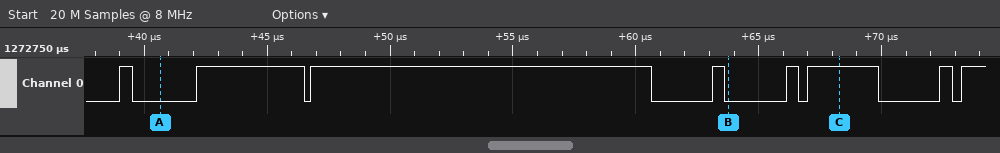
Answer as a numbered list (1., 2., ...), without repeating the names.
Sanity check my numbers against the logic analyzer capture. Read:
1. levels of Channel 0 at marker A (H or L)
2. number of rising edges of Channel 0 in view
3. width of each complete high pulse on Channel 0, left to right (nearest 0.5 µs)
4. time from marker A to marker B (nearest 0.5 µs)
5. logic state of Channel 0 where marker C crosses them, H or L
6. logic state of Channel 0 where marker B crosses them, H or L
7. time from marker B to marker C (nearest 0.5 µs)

1. Channel 0=L
2. 8
3. 0.5 µs, 4.5 µs, 14 µs, 0.5 µs, 0.5 µs, 3 µs, 0.5 µs
4. 23 µs
5. Channel 0=H
6. Channel 0=L
7. 4.5 µs
